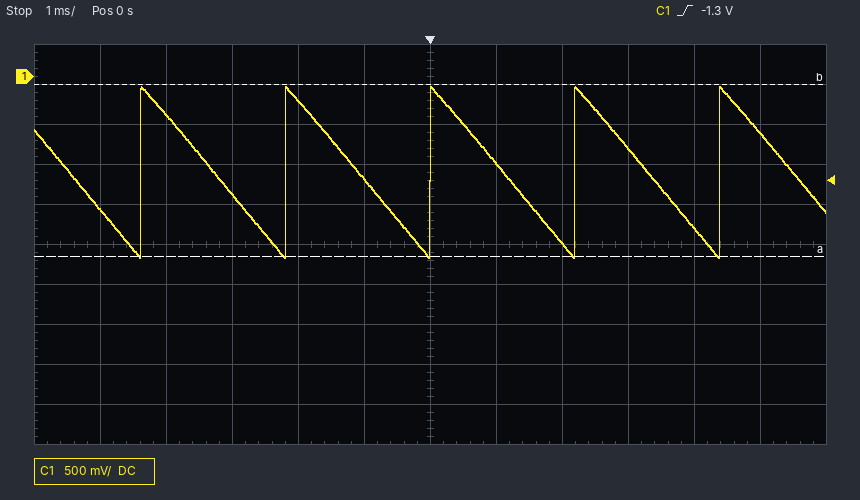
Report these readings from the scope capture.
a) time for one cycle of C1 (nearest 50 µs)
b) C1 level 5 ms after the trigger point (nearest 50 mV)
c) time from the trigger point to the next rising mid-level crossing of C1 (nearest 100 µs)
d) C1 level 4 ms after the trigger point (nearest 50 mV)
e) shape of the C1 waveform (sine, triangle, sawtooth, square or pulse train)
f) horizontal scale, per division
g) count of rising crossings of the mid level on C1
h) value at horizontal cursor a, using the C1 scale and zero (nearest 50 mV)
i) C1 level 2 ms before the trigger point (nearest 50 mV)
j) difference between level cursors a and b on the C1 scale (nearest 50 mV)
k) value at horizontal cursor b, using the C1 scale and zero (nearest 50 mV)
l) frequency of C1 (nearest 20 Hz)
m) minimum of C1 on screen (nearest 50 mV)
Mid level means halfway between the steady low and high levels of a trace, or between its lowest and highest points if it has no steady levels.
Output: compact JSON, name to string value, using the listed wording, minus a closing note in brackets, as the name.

{"time for one cycle of C1": "2.20 ms", "C1 level 5 ms after the trigger point": "-700 mV", "time from the trigger point to the next rising mid-level crossing of C1": "2.2 ms", "C1 level 4 ms after the trigger point": "-1.90 V", "shape of the C1 waveform": "sawtooth", "horizontal scale, per division": "1 ms", "count of rising crossings of the mid level on C1": "5", "value at horizontal cursor a, using the C1 scale and zero": "-2.25 V", "C1 level 2 ms before the trigger point": "-300 mV", "difference between level cursors a and b on the C1 scale": "2.15 V", "value at horizontal cursor b, using the C1 scale and zero": "-100 mV", "frequency of C1": "460 Hz", "minimum of C1 on screen": "-2.25 V"}
